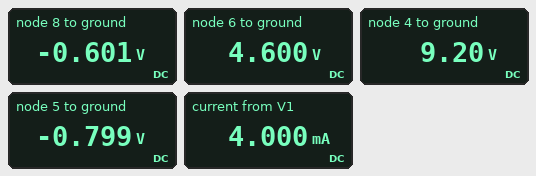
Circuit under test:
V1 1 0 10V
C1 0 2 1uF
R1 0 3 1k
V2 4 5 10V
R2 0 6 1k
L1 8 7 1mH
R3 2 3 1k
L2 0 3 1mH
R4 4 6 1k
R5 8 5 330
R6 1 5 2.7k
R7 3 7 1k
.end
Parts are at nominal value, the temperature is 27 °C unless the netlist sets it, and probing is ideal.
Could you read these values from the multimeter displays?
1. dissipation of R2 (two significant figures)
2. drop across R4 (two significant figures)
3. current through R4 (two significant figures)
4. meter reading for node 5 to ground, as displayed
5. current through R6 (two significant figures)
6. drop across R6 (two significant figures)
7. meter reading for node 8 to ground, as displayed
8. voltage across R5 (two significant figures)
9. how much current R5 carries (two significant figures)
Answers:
21 mW
4.6 V
4.6 mA
-0.799 V
4.0 mA
11 V
-0.601 V
200 mV
600 µA
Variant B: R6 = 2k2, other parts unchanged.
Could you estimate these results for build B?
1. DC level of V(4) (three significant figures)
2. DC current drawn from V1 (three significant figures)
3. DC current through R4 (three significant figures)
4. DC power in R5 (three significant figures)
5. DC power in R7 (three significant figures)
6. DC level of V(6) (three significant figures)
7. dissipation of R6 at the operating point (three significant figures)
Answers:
9.73 V
4.67 mA
4.87 mA
13.2 µW
40.1 µW
4.87 V
47.9 mW
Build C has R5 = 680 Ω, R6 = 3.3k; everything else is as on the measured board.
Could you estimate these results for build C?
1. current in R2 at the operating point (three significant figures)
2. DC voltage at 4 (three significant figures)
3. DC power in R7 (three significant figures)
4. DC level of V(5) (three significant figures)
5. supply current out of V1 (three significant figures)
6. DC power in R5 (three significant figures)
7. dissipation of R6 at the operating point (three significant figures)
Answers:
4.30 mA
8.59 V
703 µW
-1.41 V
3.46 mA
478 µW
39.4 mW
